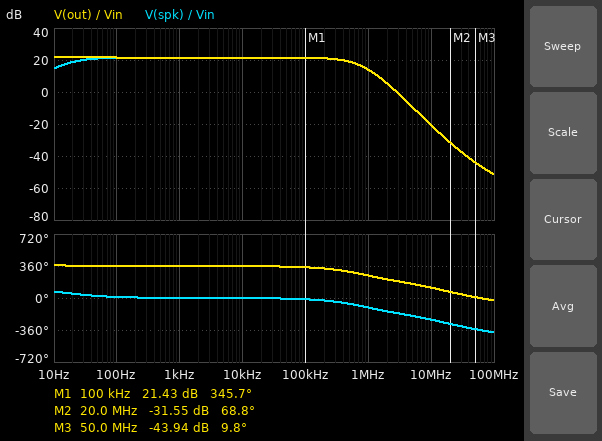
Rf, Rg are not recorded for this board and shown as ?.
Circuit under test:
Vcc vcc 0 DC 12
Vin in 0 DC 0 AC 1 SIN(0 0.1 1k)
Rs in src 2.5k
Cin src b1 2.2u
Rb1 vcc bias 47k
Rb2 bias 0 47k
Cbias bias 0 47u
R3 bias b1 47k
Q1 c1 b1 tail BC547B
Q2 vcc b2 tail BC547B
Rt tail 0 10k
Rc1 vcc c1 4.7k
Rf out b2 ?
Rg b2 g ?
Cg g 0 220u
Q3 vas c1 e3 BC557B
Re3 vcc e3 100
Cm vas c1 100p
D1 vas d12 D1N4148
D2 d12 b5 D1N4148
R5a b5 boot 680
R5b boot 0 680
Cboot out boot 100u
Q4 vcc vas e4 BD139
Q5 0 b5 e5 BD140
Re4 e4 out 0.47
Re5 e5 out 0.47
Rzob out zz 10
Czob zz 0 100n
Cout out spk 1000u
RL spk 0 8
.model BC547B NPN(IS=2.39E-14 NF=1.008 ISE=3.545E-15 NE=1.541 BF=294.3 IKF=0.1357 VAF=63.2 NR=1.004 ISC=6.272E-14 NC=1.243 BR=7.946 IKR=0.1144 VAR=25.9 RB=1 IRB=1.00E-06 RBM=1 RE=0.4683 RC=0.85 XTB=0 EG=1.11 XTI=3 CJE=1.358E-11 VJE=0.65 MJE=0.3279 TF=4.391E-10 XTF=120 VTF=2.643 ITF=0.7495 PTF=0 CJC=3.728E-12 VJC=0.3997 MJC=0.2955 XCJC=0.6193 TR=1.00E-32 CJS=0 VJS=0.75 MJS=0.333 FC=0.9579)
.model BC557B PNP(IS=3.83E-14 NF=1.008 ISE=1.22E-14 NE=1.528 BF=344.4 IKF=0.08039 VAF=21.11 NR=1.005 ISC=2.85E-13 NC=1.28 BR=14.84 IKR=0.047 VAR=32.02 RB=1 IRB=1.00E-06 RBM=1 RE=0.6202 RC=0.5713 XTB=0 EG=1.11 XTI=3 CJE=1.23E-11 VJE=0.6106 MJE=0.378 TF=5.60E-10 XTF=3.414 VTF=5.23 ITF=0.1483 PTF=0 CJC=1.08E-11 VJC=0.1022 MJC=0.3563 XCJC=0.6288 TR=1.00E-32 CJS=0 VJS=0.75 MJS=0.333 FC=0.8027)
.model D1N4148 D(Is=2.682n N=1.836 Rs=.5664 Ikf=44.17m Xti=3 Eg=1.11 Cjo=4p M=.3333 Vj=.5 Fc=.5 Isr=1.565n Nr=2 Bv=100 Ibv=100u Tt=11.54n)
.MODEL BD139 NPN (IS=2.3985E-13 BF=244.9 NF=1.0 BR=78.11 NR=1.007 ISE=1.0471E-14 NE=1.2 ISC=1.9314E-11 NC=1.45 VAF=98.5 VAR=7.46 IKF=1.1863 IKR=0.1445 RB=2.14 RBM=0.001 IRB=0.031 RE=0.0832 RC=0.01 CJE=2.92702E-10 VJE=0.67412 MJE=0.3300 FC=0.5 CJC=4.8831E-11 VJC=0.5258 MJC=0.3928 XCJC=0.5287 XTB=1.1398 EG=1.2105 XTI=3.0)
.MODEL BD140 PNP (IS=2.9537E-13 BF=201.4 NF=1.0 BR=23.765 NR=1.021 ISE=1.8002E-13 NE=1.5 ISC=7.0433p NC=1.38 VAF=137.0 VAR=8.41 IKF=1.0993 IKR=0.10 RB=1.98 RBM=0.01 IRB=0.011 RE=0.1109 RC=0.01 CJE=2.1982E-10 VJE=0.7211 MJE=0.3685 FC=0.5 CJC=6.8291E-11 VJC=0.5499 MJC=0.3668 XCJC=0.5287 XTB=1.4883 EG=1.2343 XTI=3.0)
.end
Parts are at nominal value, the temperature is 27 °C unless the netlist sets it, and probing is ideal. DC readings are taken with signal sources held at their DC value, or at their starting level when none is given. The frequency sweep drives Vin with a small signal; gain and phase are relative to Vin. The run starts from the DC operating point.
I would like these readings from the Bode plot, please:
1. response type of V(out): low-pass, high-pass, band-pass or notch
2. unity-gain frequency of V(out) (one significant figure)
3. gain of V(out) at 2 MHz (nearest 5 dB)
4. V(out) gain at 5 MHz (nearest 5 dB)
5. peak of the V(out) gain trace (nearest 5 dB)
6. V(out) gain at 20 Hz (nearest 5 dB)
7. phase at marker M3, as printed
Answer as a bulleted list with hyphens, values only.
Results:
- low-pass
- 3 MHz
- 5 dB
- -10 dB
- 20 dB
- 20 dB
- 9.8 deg
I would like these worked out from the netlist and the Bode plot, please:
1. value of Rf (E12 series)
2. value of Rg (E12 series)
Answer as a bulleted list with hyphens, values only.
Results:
- 33 kΩ
- 2.7 kΩ
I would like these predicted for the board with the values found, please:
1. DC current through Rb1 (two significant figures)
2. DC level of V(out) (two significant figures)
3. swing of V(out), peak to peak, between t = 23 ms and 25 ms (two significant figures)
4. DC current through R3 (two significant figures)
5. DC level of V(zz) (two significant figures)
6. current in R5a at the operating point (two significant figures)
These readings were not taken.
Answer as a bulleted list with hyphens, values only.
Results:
- 130 µA
- 6.0 V
- 2.4 V
- 760 nA
- 6.0 V
- 3.9 mA
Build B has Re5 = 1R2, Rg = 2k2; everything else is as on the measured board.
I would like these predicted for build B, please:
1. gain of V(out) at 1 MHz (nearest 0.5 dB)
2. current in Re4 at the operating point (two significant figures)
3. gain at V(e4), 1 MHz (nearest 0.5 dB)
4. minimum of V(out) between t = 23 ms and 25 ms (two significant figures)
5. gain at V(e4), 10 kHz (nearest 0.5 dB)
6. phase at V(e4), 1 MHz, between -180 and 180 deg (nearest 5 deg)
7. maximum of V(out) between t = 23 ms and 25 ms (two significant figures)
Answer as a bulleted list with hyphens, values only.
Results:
- 13.5 dB
- 27 mA
- 14.0 dB
- 4.6 V
- 23.5 dB
- -110 deg
- 7.4 V
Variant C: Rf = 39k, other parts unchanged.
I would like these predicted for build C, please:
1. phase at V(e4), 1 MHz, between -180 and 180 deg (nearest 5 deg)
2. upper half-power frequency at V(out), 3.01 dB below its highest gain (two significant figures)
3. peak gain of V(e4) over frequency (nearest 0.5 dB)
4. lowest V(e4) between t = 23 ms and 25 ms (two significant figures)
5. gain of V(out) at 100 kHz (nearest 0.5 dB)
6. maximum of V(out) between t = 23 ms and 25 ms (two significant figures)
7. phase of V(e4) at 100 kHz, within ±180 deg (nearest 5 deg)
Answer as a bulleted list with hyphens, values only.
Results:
- -110 deg
- 420 kHz
- 23.0 dB
- 4.6 V
- 22.5 dB
- 7.4 V
- -15 deg
